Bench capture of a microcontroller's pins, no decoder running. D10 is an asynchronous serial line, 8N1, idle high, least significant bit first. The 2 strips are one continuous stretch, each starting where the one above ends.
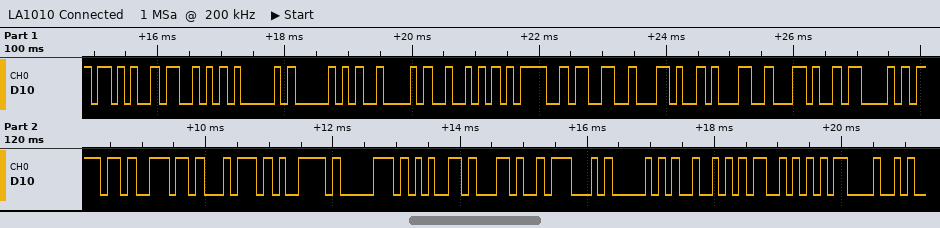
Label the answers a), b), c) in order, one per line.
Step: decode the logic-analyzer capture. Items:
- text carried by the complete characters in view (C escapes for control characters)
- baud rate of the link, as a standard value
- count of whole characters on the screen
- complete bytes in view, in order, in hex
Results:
a) "+SAPBR=3,1,Contype,GPRS\r"
b) 9600 baud
c) 24
d) 2B 53 41 50 42 52 3D 33 2C 31 2C 43 6F 6E 74 79 70 65 2C 47 50 52 53 0D
